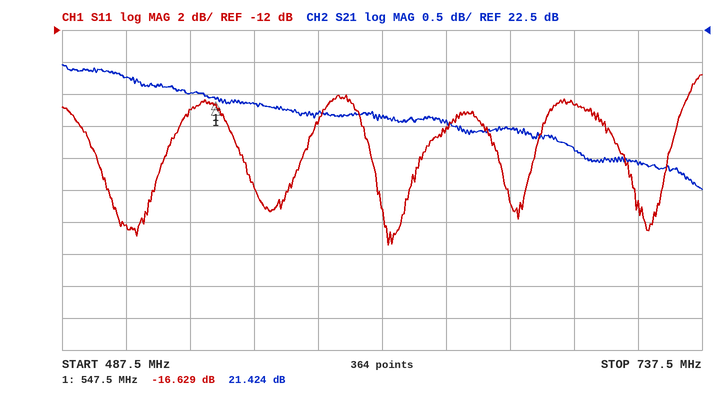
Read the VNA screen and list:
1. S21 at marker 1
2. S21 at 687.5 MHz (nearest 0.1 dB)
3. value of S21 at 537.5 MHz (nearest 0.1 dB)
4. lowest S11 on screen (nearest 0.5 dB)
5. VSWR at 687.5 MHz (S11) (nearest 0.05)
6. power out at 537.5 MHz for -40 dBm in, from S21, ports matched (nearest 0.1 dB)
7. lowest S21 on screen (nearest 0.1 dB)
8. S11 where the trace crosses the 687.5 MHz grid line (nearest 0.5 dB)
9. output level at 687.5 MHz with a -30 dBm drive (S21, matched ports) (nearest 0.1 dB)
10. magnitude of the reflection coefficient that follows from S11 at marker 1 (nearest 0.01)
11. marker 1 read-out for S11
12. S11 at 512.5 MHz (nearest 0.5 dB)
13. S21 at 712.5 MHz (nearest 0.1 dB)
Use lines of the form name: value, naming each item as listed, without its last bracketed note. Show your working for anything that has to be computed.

S21 at marker 1: 21.424 dB
S21 at 687.5 MHz: 20.6 dB
value of S21 at 537.5 MHz: 21.5 dB
lowest S11 on screen: -25.5 dB
VSWR at 687.5 MHz (S11): |Γ| = 10^(-16.5/20) = 0.1496; VSWR = (1 + 0.1496)/(1 − 0.1496) ≈ 1.35
power out at 537.5 MHz for -40 dBm in, from S21, ports matched: -40 dBm + (21.5 dB) = -18.5 dBm
lowest S21 on screen: 20.0 dB
S11 where the trace crosses the 687.5 MHz grid line: -16.5 dB
output level at 687.5 MHz with a -30 dBm drive (S21, matched ports): -30 dBm + (20.6 dB) = -9.4 dBm
magnitude of the reflection coefficient that follows from S11 at marker 1: 10^(-16.629/20) ≈ 0.15
marker 1 read-out for S11: -16.629 dB
S11 at 512.5 MHz: -24.0 dB
S21 at 712.5 MHz: 20.4 dB
